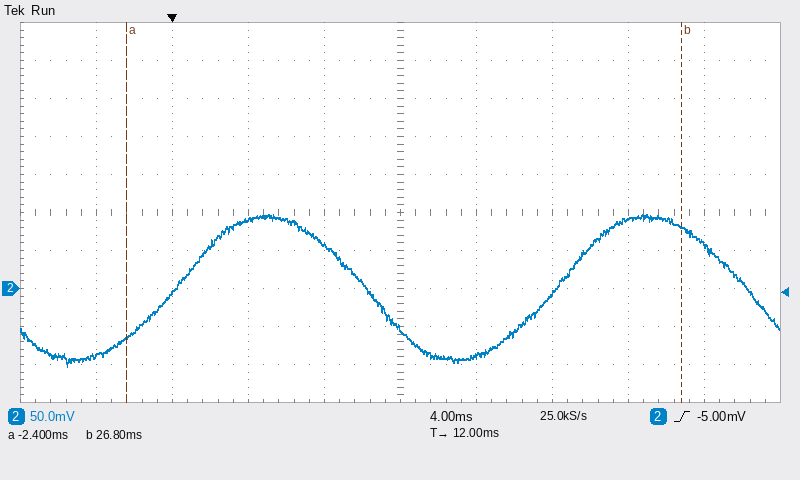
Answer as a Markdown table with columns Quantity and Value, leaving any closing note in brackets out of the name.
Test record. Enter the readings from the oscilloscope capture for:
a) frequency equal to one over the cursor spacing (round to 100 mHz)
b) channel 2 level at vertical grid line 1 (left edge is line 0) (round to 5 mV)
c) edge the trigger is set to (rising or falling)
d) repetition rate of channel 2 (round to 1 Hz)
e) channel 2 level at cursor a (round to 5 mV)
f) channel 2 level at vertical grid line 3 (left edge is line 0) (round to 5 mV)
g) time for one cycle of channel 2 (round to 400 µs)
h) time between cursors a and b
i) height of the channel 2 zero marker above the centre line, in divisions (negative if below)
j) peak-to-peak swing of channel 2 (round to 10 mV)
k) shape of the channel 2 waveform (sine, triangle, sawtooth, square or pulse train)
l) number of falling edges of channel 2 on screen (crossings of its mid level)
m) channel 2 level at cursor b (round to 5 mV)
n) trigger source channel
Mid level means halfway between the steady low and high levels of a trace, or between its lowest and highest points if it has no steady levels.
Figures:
| Quantity | Value |
|---|---|
| frequency equal to one over the cursor spacing | 34.2 Hz |
| channel 2 level at vertical grid line 1 (left edge is line 0) | -90 mV |
| edge the trigger is set to | rising |
| repetition rate of channel 2 | 50 Hz |
| channel 2 level at cursor a | -65 mV |
| channel 2 level at vertical grid line 3 (left edge is line 0) | 90 mV |
| time for one cycle of channel 2 | 20.0 ms |
| time between cursors a and b | 29.2 ms |
| height of the channel 2 zero marker above the centre line, in divisions | -2.0 div |
| peak-to-peak swing of channel 2 | 200 mV |
| shape of the channel 2 waveform | sine |
| number of falling edges of channel 2 on screen | 2 |
| channel 2 level at cursor b | 80 mV |
| trigger source channel | channel 2 |
